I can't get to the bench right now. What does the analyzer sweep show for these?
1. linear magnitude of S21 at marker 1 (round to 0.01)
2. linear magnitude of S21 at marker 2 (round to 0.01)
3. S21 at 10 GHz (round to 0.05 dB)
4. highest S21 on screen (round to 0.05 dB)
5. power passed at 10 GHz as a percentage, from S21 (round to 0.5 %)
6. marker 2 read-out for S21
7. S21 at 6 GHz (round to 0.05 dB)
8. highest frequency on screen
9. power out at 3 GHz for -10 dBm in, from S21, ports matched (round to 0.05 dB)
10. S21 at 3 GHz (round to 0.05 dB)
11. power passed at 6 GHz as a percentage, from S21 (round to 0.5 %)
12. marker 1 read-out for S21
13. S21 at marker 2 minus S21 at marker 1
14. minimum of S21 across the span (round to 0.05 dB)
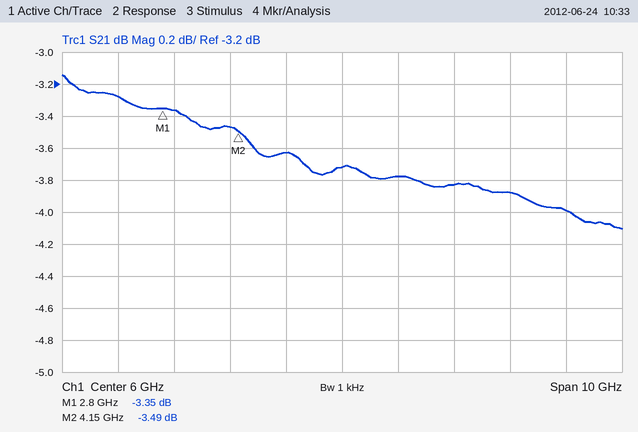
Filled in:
0.68
0.67
-4.00 dB
-3.15 dB
40.0 %
-3.49 dB
-3.70 dB
11 GHz
-13.35 dBm
-3.35 dB
42.5 %
-3.35 dB
-0.14 dB
-4.10 dB
